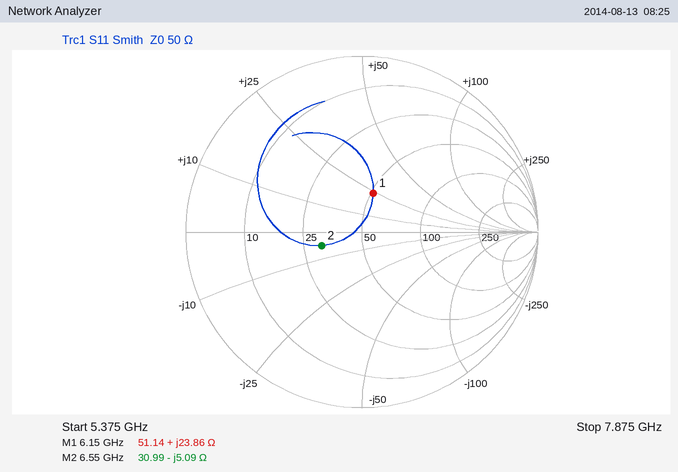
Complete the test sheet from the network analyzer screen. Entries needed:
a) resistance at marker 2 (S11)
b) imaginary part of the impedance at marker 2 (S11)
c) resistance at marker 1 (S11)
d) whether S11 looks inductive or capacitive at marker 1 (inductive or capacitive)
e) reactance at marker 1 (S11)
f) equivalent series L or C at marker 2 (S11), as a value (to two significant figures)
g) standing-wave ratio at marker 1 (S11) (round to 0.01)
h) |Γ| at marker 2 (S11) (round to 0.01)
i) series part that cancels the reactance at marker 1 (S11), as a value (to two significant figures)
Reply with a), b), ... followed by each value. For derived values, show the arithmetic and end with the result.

a) 30.99 Ω
b) -5.09 Ω
c) 51.14 Ω
d) inductive
e) +23.86 Ω
f) C = 1/(2π × 6.55 GHz × 5.09 Ω) ≈ 4.8 pF
g) 1.60
h) 0.24
i) C = 1/(2π × 6.15 GHz × 23.86 Ω) ≈ 1.1 pF
